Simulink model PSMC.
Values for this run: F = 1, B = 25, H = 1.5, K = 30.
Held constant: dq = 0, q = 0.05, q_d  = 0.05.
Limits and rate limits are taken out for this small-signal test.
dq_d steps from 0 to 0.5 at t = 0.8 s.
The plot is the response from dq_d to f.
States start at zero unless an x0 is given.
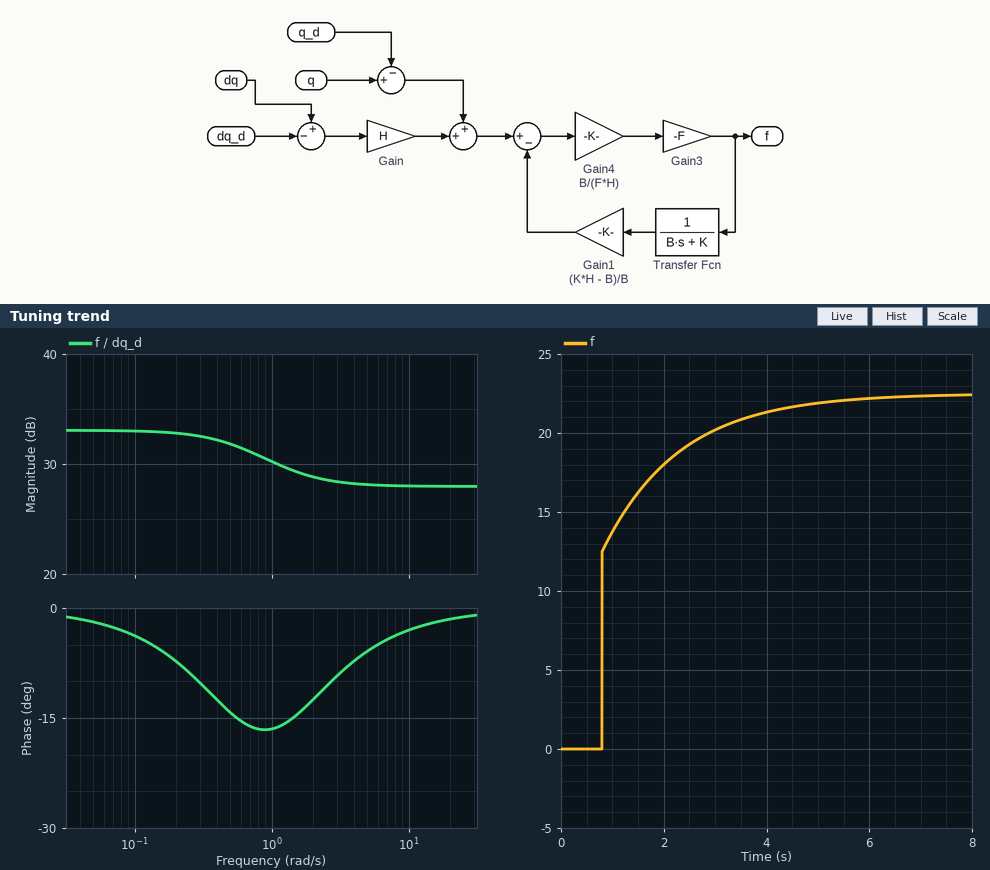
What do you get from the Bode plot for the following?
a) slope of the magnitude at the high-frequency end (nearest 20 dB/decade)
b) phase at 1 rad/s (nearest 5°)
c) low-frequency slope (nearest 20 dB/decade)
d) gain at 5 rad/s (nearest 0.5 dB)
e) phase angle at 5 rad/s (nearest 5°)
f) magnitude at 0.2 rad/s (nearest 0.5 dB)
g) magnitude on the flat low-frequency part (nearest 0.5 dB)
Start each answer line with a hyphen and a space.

- 0 dB/decade
- -15°
- 0 dB/decade
- 28.0 dB
- -5°
- 33.0 dB
- 33.0 dB
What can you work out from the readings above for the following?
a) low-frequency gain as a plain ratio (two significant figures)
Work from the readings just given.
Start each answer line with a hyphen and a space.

- 45
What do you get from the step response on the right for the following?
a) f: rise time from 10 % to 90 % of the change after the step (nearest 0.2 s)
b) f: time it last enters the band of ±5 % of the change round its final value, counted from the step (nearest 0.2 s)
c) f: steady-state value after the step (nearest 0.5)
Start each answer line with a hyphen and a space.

- 2.2 s
- 3.2 s
- 22.5
